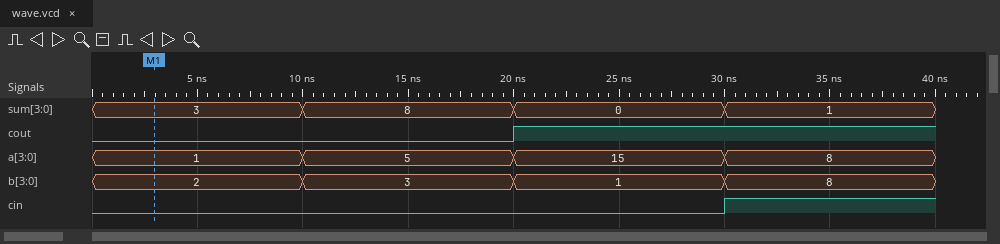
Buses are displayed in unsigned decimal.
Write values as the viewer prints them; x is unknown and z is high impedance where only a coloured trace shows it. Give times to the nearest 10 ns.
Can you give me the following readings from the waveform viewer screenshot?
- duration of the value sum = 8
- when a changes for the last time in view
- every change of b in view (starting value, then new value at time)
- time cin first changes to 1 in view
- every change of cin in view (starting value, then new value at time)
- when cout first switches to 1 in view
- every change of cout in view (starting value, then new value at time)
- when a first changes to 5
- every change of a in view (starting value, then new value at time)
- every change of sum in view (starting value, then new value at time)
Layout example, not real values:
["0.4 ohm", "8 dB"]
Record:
["10 ns", "30 ns", "2, 3 at 10 ns, 1 at 20 ns, 8 at 30 ns", "30 ns", "0, 1 at 30 ns", "20 ns", "0, 1 at 20 ns", "10 ns", "1, 5 at 10 ns, 15 at 20 ns, 8 at 30 ns", "3, 8 at 10 ns, 0 at 20 ns, 1 at 30 ns"]
